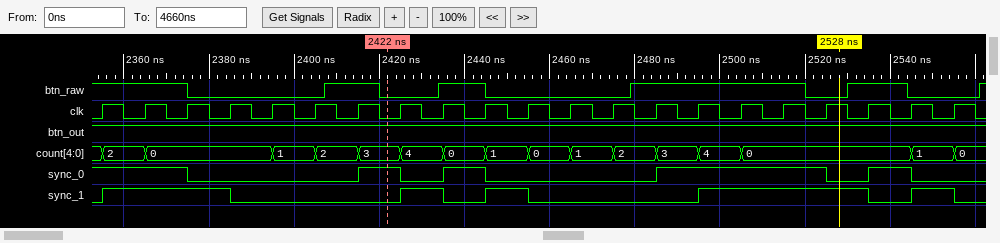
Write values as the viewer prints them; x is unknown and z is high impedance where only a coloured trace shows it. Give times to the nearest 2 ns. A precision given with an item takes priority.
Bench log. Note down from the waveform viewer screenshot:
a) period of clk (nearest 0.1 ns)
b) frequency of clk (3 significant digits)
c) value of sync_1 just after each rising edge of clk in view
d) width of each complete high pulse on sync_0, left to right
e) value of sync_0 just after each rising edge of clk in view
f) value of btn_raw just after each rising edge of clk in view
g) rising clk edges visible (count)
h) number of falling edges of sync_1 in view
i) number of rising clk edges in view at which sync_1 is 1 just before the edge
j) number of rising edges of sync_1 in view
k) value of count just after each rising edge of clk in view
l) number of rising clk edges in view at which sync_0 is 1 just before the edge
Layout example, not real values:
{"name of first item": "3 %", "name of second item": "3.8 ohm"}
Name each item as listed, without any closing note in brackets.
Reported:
{"period of clk": "10 ns", "frequency of clk": "100 MHz", "value of sync_1 just after each rising edge of clk in view": "1 1 1 0 0 0 0 1 0 1 0 0 0 0 1 1 1 1 0 1 0", "width of each complete high pulse on sync_0, left to right": "10 ns, 10 ns, 40 ns, 10 ns", "value of sync_0 just after each rising edge of clk in view": "1 1 0 0 0 0 1 0 1 0 0 0 0 1 1 1 1 0 1 0 0", "value of btn_raw just after each rising edge of clk in view": "1 1 0 0 0 0 1 0 1 0 0 0 0 1 1 1 1 0 1 0 0", "rising clk edges visible": "21", "number of falling edges of sync_1 in view": "5", "number of rising clk edges in view at which sync_1 is 1 just before the edge": "10", "number of rising edges of sync_1 in view": "5", "value of count just after each rising edge of clk in view": "2, 0, 0, 0, 1, 2, 3, 4, 0, 1, 0, 1, 2, 3, 4, 0, 0, 0, 0, 1, 0", "number of rising clk edges in view at which sync_0 is 1 just before the edge": "10"}
